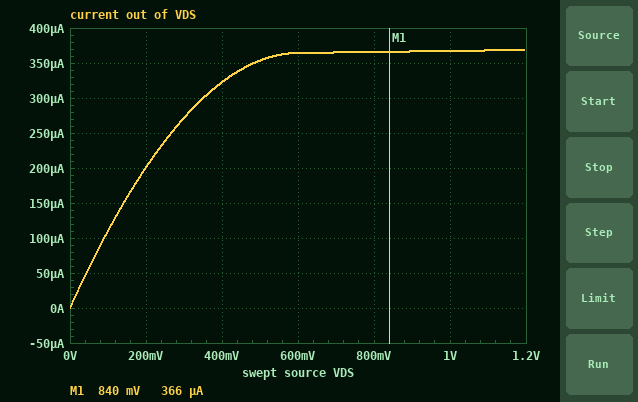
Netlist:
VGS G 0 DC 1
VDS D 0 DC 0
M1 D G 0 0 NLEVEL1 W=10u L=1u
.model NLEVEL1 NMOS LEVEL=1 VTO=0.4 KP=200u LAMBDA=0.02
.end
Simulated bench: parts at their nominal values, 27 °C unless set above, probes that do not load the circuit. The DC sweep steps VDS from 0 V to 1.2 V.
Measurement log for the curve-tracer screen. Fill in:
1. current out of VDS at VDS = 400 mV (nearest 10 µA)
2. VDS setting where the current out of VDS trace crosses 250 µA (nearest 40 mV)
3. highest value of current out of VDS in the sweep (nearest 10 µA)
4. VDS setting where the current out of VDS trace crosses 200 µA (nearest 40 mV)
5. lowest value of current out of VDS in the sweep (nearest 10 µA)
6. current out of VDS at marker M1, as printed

320 µA
280 mV
370 µA
200 mV
0 A
366 µA
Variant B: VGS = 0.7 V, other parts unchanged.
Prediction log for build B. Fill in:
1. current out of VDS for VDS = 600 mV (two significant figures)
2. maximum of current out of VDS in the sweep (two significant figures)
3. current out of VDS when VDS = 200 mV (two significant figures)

91 µA
92 µA
80 µA
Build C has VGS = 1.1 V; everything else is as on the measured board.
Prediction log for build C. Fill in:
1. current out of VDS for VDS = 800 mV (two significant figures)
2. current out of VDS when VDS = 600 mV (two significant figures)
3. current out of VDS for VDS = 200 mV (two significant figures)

500 µA
490 µA
240 µA
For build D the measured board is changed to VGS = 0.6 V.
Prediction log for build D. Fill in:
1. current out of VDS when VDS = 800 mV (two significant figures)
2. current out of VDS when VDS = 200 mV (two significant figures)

41 µA
40 µA
